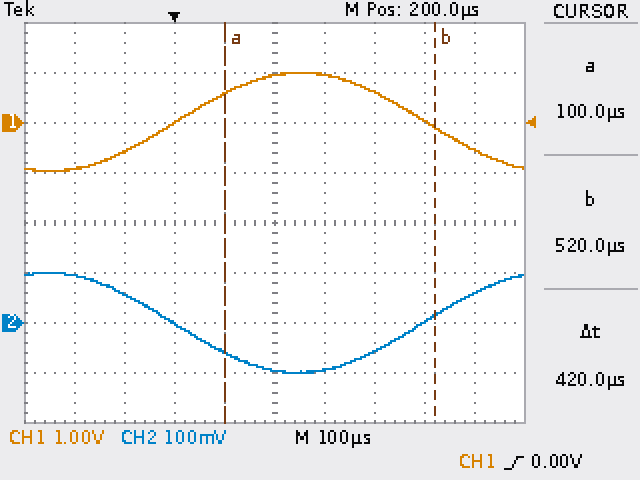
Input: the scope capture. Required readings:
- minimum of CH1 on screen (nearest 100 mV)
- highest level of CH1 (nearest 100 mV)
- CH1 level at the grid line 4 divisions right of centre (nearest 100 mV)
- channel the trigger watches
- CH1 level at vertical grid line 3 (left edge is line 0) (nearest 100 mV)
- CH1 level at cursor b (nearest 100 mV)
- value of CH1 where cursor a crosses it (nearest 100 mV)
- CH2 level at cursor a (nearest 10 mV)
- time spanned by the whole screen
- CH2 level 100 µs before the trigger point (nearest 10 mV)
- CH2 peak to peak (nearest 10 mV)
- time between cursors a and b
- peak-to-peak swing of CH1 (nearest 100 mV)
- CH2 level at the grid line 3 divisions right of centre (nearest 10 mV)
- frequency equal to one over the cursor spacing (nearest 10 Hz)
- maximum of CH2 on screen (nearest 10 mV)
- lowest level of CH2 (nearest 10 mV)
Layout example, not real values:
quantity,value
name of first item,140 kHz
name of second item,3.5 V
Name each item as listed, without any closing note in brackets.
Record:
quantity,value
minimum of CH1 on screen,-1.0 V
highest level of CH1,1.0 V
CH1 level at the grid line 4 divisions right of centre,-500 mV
channel the trigger watches,CH1
CH1 level at vertical grid line 3 (left edge is line 0),0.0 V
CH1 level at cursor b,-100 mV
value of CH1 where cursor a crosses it,600 mV
CH2 level at cursor a,-60 mV
time spanned by the whole screen,1 ms
CH2 level 100 µs before the trigger point,60 mV
CH2 peak to peak,200 mV
time between cursors a and b,420 µs
peak-to-peak swing of CH1,2.0 V
CH2 level at the grid line 3 divisions right of centre,0 mV
frequency equal to one over the cursor spacing,2.38 kHz
maximum of CH2 on screen,100 mV
lowest level of CH2,-100 mV
